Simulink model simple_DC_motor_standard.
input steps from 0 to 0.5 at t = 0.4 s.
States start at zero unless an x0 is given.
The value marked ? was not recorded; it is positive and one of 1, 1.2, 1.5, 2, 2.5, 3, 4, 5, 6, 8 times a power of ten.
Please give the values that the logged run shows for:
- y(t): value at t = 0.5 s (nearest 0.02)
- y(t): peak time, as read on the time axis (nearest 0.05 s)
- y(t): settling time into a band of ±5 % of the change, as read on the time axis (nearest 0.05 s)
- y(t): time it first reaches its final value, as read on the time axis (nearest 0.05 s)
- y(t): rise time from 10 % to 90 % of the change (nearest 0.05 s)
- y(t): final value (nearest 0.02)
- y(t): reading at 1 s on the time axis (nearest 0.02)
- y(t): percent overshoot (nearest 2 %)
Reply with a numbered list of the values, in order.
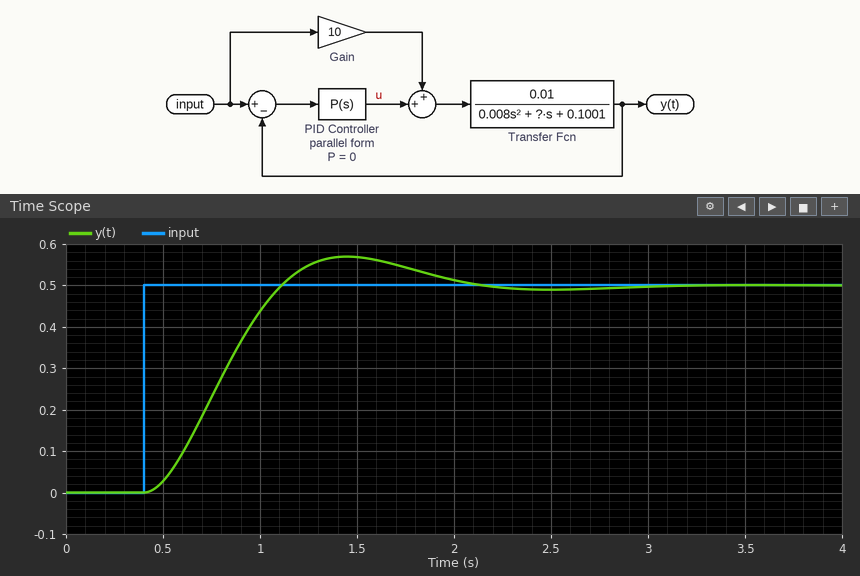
1. 0.02
2. 1.45 s
3. 1.90 s
4. 1.10 s
5. 0.50 s
6. 0.50
7. 0.44
8. 14 %
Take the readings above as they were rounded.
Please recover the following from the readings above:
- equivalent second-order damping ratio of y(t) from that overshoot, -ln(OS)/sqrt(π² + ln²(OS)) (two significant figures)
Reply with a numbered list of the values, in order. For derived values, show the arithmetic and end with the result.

1. ln(0.14) = -1.966; 1.966 / sqrt(9.870 + 3.866) = 0.53
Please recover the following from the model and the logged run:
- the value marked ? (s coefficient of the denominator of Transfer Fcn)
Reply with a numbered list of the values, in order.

1. 0.03
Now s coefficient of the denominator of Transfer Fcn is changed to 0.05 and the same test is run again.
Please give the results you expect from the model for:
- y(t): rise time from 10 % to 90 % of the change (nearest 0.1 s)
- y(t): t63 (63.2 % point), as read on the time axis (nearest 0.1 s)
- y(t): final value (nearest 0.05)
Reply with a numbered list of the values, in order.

1. 0.8 s
2. 1.0 s
3. 0.50
